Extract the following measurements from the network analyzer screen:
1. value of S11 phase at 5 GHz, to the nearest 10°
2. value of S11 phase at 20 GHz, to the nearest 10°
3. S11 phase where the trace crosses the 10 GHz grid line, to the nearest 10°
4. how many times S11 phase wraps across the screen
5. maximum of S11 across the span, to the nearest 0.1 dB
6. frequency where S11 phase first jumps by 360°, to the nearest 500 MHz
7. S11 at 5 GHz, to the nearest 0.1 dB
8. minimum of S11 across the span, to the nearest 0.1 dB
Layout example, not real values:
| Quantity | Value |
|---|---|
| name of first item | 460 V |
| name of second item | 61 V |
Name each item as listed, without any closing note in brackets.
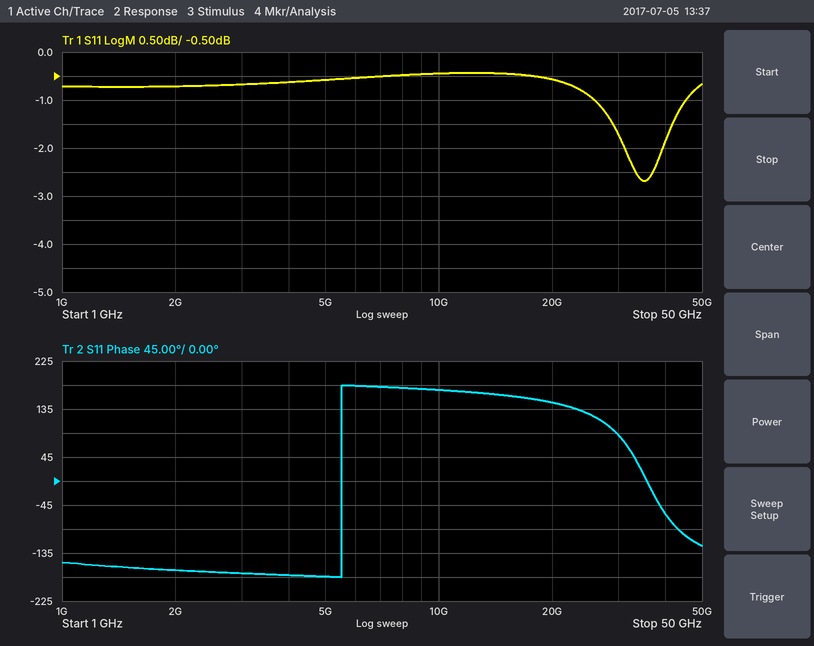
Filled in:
| Quantity | Value |
|---|---|
| value of S11 phase at 5 GHz, to the nearest 10° | -180° |
| value of S11 phase at 20 GHz, to the nearest 10° | 150° |
| S11 phase where the trace crosses the 10 GHz grid line, to the nearest 10° | 170° |
| how many times S11 phase wraps across the screen | 1 |
| maximum of S11 across the span, to the nearest 0.1 dB | -0.4 dB |
| frequency where S11 phase first jumps by 360°, to the nearest 500 MHz | 5.5 GHz |
| S11 at 5 GHz, to the nearest 0.1 dB | -0.6 dB |
| minimum of S11 across the span, to the nearest 0.1 dB | -2.7 dB |
